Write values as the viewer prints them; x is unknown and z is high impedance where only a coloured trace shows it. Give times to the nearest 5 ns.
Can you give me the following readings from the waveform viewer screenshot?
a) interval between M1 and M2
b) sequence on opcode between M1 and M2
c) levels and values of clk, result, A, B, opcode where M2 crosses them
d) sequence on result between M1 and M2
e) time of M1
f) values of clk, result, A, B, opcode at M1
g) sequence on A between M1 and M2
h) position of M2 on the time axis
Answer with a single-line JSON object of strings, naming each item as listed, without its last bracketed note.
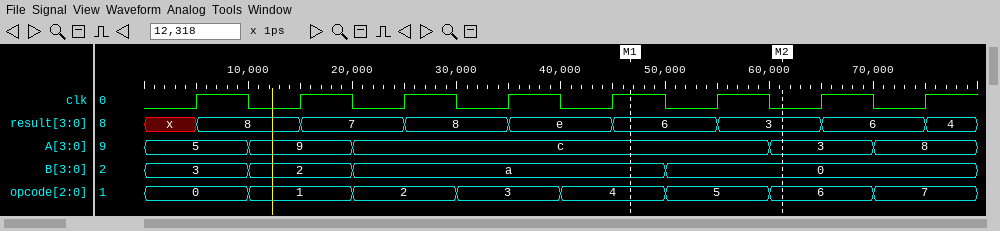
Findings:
{"interval between M1 and M2": "15 ns", "sequence on opcode between M1 and M2": "4, 5, 6", "levels and values of clk, result, A, B, opcode where M2 crosses them": "clk=0, result=3, A=3, B=0, opcode=6", "sequence on result between M1 and M2": "6, 3", "time of M1": "45 ns", "values of clk, result, A, B, opcode at M1": "clk=1, result=6, A=c, B=a, opcode=4", "sequence on A between M1 and M2": "c, 3", "position of M2 on the time axis": "60 ns"}
